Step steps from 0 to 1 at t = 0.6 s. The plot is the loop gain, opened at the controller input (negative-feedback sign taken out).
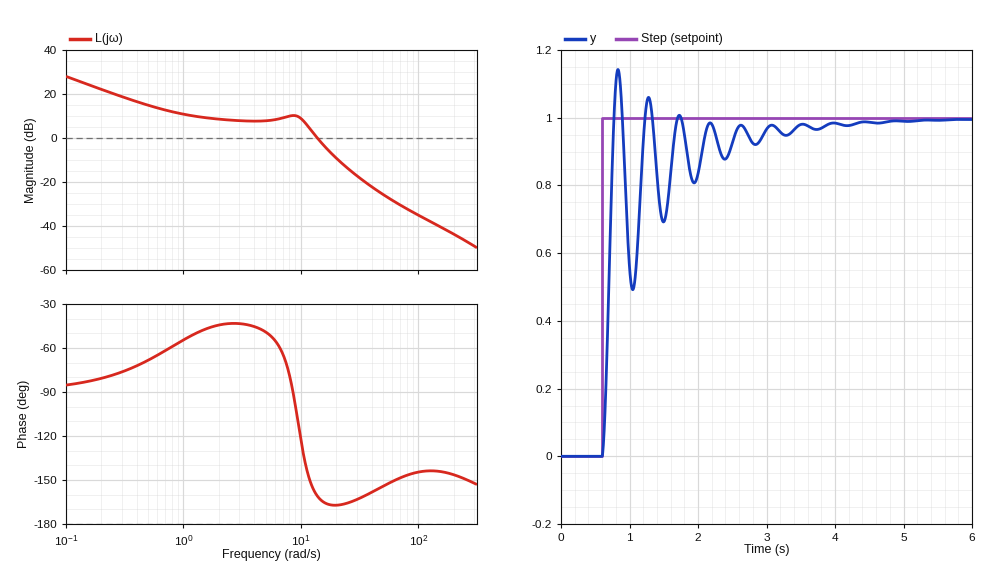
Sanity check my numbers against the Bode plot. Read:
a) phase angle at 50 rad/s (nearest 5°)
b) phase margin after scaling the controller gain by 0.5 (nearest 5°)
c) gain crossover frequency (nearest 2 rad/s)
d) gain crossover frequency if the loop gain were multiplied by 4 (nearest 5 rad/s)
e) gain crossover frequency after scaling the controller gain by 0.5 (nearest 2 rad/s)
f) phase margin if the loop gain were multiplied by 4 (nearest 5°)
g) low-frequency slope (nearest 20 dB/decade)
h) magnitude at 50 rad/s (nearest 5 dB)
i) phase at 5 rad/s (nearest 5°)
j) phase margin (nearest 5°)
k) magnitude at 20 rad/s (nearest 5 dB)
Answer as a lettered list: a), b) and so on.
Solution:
a) -155°
b) 35°
c) 14 rad/s
d) 25 rad/s
e) 12 rad/s
f) 15°
g) -20 dB/decade
h) -25 dB
i) -50°
j) 20°
k) -10 dB
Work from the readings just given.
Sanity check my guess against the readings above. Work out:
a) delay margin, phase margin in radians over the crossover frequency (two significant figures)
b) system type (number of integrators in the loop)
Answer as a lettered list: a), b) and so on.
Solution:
a) 0.025 s
b) 1
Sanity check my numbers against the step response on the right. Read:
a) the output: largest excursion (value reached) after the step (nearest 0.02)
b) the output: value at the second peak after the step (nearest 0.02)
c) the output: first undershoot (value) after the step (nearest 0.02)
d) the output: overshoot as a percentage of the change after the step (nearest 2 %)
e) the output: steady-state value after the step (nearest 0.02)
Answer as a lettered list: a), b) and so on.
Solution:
a) 1.14
b) 1.06
c) 0.50
d) 14 %
e) 1.00
